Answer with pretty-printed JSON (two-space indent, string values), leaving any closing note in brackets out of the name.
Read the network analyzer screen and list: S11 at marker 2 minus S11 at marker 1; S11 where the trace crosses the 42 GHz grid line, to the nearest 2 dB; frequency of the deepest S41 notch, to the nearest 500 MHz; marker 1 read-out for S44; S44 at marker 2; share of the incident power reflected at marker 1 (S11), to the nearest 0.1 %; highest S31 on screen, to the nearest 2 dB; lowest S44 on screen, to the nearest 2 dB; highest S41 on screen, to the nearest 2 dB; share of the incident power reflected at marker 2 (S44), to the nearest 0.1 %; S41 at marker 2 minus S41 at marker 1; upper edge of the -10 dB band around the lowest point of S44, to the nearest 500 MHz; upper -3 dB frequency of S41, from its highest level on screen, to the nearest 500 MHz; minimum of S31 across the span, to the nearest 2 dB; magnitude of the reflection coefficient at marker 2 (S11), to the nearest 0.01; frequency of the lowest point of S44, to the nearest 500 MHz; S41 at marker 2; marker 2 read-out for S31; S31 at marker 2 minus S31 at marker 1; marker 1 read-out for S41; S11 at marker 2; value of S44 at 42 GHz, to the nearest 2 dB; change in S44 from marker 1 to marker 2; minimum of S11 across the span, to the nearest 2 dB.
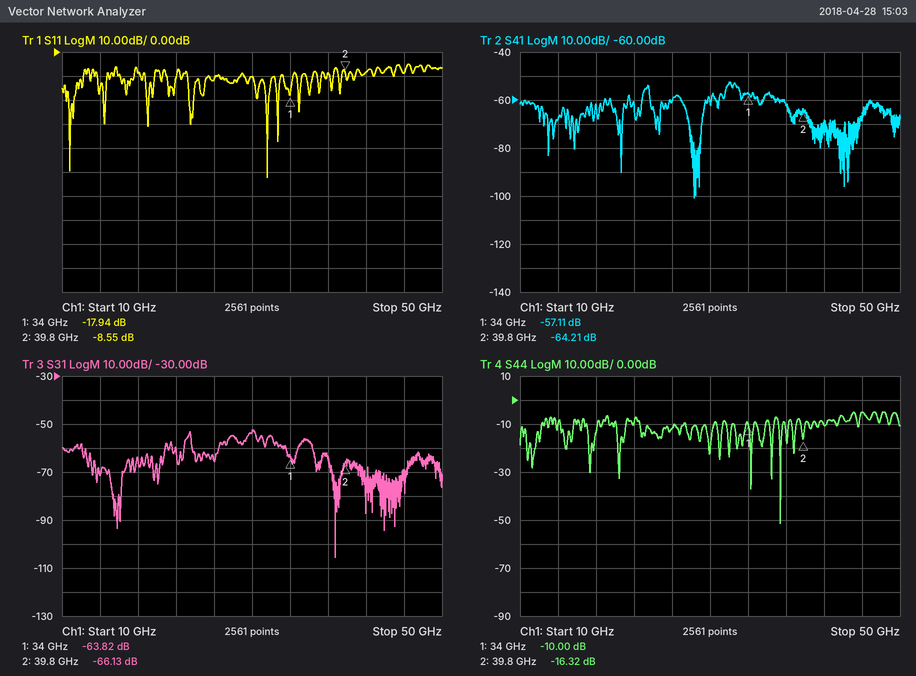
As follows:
{
  "S11 at marker 2 minus S11 at marker 1": "9.39 dB",
  "S11 where the trace crosses the 42 GHz grid line, to the nearest 2 dB": "-8 dB",
  "frequency of the deepest S41 notch, to the nearest 500 MHz": "28.5 GHz",
  "marker 1 read-out for S44": "-10.00 dB",
  "S44 at marker 2": "-16.32 dB",
  "share of the incident power reflected at marker 1 (S11), to the nearest 0.1 %": "1.6 %",
  "highest S31 on screen, to the nearest 2 dB": "-52 dB",
  "lowest S44 on screen, to the nearest 2 dB": "-52 dB",
  "highest S41 on screen, to the nearest 2 dB": "-52 dB",
  "share of the incident power reflected at marker 2 (S44), to the nearest 0.1 %": "2.3 %",
  "S41 at marker 2 minus S41 at marker 1": "-7.10 dB",
  "upper edge of the -10 dB band around the lowest point of S44, to the nearest 500 MHz": "37.5 GHz",
  "upper -3 dB frequency of S41, from its highest level on screen, to the nearest 500 MHz": "33.0 GHz",
  "minimum of S31 across the span, to the nearest 2 dB": "-106 dB",
  "magnitude of the reflection coefficient at marker 2 (S11), to the nearest 0.01": "0.37",
  "frequency of the lowest point of S44, to the nearest 500 MHz": "37.5 GHz",
  "S41 at marker 2": "-64.21 dB",
  "marker 2 read-out for S31": "-66.13 dB",
  "S31 at marker 2 minus S31 at marker 1": "-2.31 dB",
  "marker 1 read-out for S41": "-57.11 dB",
  "S11 at marker 2": "-8.55 dB",
  "value of S44 at 42 GHz, to the nearest 2 dB": "-10 dB",
  "change in S44 from marker 1 to marker 2": "-6.32 dB",
  "minimum of S11 across the span, to the nearest 2 dB": "-52 dB"
}
